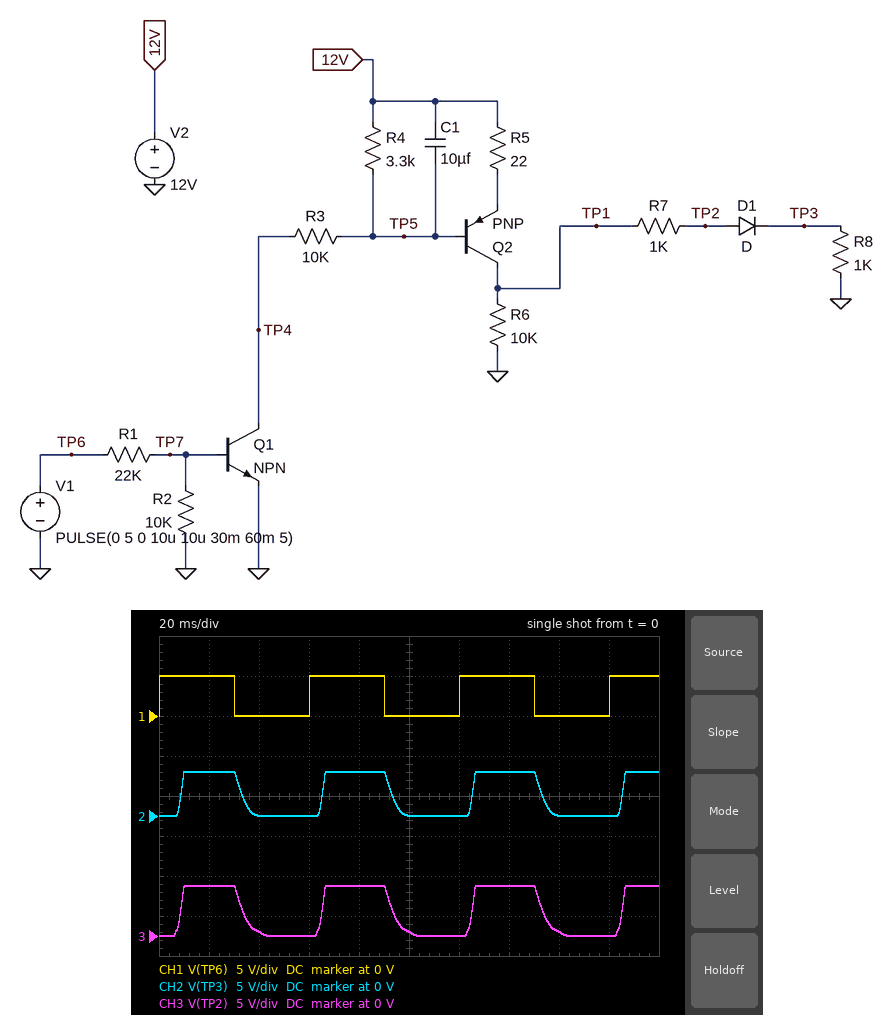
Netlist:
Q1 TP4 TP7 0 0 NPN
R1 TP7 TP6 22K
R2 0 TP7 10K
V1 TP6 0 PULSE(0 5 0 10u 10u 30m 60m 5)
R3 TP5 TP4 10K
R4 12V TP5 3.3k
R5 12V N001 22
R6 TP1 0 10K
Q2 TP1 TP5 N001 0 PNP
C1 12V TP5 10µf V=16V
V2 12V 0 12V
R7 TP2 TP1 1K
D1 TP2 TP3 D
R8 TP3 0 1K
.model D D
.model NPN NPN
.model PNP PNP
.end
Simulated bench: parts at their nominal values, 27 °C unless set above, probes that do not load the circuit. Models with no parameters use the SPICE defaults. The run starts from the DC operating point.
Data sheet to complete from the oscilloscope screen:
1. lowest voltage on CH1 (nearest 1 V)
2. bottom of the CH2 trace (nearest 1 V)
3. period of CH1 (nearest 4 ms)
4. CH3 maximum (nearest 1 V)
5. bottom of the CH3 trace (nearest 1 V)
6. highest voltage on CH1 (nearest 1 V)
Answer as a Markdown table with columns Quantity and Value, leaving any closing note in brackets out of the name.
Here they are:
| Quantity | Value |
|---|---|
| lowest voltage on CH1 | 0 V |
| bottom of the CH2 trace | 0 V |
| period of CH1 | 60 ms |
| CH3 maximum | 6 V |
| bottom of the CH3 trace | 0 V |
| highest voltage on CH1 | 5 V |
